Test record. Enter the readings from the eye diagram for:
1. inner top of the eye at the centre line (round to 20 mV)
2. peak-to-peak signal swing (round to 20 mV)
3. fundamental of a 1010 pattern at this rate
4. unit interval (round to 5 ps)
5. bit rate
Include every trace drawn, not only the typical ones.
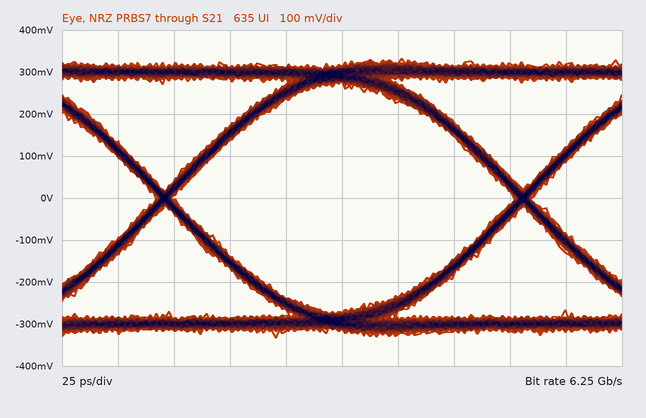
280 mV
660 mV
3.125 GHz
160 ps
6.25 Gb/s
